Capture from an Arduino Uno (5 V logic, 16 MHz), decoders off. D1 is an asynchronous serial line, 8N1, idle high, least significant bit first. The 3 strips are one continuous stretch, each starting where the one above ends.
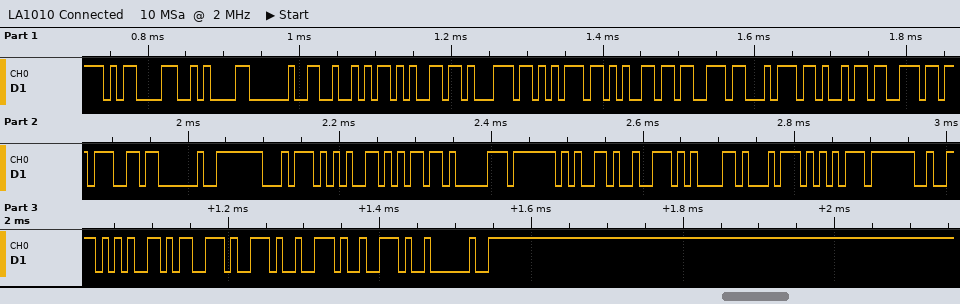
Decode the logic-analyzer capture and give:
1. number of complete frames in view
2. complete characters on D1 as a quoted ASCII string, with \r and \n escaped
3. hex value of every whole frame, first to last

30
"\r\n Requesting temperatures... "
0D 0A 20 52 65 71 75 65 73 74 69 6E 67 20 74 65 6D 70 65 72 61 74 75 72 65 73 2E 2E 2E 20
